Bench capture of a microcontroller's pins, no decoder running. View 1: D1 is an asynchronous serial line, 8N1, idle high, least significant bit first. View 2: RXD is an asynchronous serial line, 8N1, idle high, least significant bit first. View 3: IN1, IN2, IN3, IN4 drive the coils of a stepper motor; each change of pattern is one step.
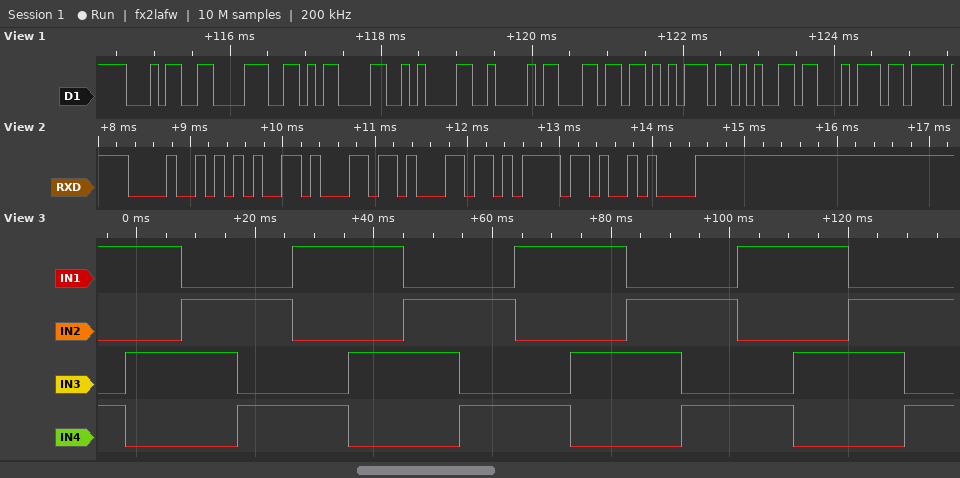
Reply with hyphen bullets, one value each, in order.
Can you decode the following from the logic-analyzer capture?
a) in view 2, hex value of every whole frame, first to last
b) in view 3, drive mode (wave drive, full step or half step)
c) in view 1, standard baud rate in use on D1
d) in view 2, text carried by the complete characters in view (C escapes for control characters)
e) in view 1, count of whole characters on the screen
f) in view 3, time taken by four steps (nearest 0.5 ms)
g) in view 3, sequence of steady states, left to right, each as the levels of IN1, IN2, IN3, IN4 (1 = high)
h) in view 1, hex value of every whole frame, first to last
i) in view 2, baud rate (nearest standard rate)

- 48 65 6C 6C 6F 0A
- full step
- 9600 baud
- "Hello\n"
- 9
- 37.5 ms
- 1001 1010 0110 0101 1001 1010 0110 0101 1001 1010 0110 0101 1001 1010 0110 0101
- 0x34 0x38 0x0D 0x0A 0x42 0x6C 0x75 0x65 0x74
- 9600 baud
